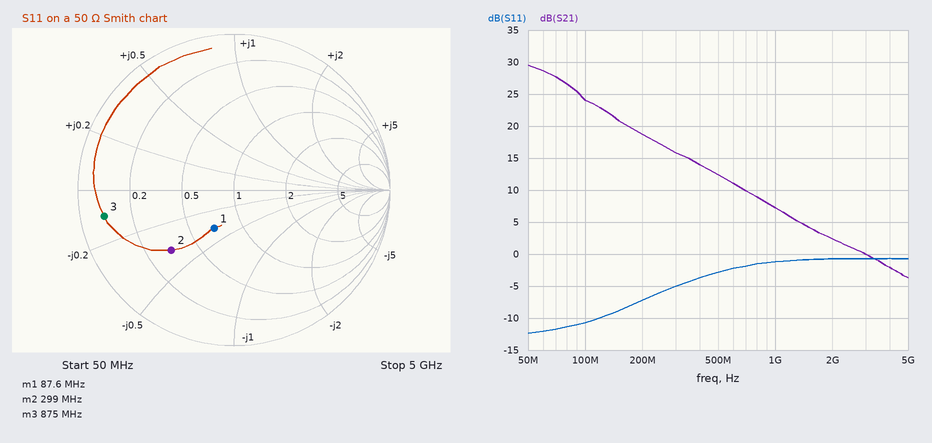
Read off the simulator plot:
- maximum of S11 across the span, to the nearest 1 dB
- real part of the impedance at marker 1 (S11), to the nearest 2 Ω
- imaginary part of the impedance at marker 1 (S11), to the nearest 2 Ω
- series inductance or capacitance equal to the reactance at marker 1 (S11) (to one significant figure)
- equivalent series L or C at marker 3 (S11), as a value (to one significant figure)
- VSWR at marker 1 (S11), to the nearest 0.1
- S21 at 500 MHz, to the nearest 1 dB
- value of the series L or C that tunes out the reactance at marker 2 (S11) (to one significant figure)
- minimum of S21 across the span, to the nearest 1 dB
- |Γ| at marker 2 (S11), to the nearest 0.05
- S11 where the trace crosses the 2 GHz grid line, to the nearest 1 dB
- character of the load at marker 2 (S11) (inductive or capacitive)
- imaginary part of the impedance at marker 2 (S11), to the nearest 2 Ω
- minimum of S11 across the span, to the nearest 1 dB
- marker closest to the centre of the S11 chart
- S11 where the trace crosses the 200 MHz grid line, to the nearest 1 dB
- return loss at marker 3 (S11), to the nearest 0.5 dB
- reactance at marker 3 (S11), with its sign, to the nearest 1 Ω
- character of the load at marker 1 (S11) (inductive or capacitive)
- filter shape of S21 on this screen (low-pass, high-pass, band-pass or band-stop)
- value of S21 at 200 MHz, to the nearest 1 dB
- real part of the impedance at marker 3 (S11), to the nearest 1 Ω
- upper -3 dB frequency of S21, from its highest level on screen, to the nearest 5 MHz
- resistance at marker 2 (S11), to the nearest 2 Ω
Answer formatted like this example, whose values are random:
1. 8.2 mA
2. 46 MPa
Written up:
1. -1 dB
2. 34 Ω
3. -18 Ω
4. 100 pF
5. 40 pF
6. 1.8
7. 12 dB
8. 10 nH
9. -4 dB
10. 0.55
11. -1 dB
12. capacitive
13. -18 Ω
14. -12 dB
15. marker 1
16. -7 dB
17. 1.5 dB
18. -5 Ω
19. capacitive
20. low-pass
21. 19 dB
22. 4 Ω
23. 80 MHz
24. 16 Ω
